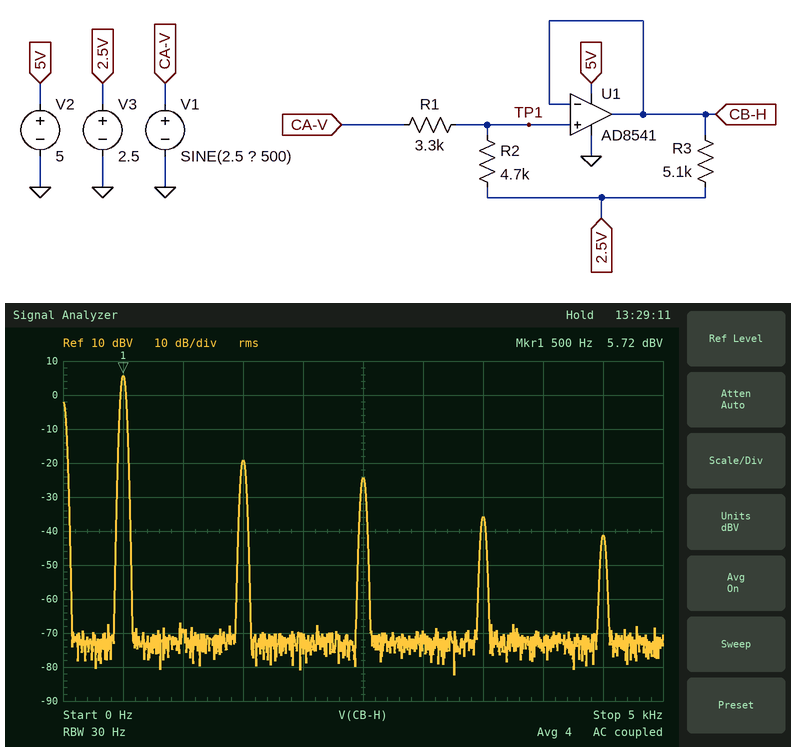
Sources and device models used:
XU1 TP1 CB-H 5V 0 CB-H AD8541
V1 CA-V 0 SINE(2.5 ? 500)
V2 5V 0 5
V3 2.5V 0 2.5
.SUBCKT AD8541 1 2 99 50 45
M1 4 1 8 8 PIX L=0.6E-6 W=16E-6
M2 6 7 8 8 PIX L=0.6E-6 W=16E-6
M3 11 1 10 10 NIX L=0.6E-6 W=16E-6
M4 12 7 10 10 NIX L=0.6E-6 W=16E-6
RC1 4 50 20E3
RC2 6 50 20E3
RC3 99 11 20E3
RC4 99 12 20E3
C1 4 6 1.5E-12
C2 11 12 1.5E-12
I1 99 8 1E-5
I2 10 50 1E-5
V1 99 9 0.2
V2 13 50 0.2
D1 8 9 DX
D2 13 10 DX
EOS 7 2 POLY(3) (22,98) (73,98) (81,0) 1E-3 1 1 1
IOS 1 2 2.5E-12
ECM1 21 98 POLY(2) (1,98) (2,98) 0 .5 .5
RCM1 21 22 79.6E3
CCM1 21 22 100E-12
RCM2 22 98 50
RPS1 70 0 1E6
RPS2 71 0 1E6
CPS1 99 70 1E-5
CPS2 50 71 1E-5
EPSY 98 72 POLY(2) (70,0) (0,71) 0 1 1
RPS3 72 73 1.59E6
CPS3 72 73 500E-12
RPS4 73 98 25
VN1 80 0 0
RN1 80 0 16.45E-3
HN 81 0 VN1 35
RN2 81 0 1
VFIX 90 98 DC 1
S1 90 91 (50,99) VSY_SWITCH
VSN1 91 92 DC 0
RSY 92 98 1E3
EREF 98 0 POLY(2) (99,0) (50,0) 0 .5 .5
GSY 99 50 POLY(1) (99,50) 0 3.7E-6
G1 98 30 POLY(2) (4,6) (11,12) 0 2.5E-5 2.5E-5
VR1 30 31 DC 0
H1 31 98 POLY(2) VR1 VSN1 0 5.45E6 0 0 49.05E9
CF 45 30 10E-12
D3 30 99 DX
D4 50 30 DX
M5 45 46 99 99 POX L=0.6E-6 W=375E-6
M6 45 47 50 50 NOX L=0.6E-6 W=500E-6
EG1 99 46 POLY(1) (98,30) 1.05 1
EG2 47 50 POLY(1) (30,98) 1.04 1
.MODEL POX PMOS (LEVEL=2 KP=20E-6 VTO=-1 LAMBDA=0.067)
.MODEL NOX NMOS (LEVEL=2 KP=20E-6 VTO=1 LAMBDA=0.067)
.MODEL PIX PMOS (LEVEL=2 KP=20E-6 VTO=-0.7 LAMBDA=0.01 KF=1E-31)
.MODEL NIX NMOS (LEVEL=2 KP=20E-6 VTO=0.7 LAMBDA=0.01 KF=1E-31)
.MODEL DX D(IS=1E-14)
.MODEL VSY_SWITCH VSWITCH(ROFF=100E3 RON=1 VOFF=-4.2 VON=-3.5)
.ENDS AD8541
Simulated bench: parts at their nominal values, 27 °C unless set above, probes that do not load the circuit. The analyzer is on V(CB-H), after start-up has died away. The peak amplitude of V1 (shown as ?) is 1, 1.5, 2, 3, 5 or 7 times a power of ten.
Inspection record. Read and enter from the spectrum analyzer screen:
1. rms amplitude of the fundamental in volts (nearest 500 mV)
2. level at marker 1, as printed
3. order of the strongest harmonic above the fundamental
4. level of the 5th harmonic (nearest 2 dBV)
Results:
2.0 V
5.72 dBV
3
-24 dBV
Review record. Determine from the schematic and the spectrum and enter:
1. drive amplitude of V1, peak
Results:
5 V
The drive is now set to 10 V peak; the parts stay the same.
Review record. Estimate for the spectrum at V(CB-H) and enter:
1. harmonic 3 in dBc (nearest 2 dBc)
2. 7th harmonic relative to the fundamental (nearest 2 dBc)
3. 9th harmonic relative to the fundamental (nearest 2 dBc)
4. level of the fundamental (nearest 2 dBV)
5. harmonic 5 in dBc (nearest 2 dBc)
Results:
-12 dBc
-44 dBc
-34 dBc
6 dBV
-22 dBc
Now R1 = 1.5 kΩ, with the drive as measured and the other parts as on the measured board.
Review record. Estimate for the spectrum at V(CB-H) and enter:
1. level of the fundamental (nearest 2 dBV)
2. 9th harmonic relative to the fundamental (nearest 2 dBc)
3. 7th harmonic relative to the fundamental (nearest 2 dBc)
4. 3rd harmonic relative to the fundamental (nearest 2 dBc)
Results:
6 dBV
-58 dBc
-32 dBc
-16 dBc
